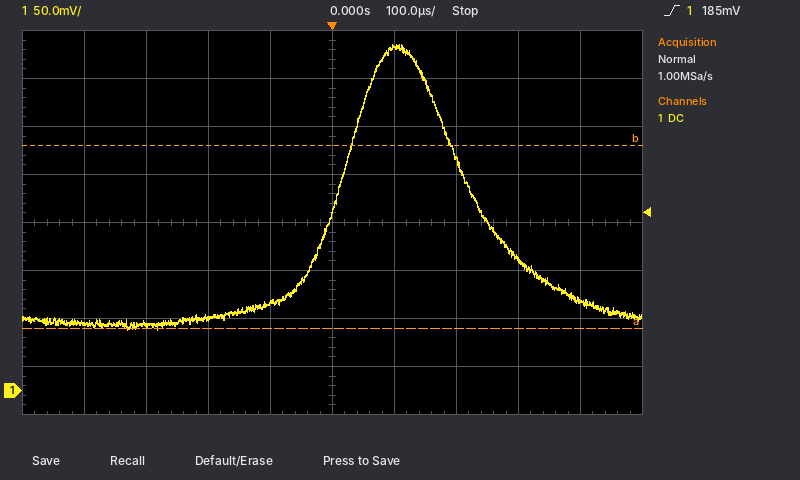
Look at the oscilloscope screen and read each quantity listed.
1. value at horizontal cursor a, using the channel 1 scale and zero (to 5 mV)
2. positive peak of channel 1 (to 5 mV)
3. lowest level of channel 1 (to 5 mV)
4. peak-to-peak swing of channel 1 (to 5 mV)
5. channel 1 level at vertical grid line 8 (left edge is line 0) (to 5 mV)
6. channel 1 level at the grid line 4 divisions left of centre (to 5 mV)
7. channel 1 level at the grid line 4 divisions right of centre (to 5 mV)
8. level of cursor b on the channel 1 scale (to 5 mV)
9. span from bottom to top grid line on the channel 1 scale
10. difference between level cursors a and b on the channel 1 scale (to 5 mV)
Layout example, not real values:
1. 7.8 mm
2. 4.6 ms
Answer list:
1. 65 mV
2. 360 mV
3. 65 mV
4. 295 mV
5. 135 mV
6. 70 mV
7. 95 mV
8. 255 mV
9. 400 mV
10. 190 mV
